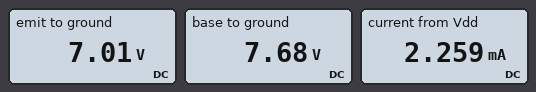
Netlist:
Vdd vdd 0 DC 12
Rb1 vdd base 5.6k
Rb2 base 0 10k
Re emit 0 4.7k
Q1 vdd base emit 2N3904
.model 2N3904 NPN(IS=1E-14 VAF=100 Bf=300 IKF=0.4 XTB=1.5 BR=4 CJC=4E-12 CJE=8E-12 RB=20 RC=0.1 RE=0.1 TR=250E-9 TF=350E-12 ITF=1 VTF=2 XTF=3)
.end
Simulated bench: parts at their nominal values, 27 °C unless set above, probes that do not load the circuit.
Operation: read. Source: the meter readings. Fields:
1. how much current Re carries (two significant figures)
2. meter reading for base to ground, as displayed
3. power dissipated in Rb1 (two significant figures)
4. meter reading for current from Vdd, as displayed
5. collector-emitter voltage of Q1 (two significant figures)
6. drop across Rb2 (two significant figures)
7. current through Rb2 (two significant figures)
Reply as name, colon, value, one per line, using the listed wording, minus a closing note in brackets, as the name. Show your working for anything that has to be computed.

how much current Re carries: (7.01 V) / 4.7 kΩ = 1.5 mA
meter reading for base to ground, as displayed: 7.68 V
power dissipated in Rb1: (12 V - 7.68 V)^2 / 5.6 kΩ = 3.3 mW
meter reading for current from Vdd, as displayed: 2.259 mA
collector-emitter voltage of Q1: 12 V - 7.01 V = 5.0 V
drop across Rb2: 7.68 V = 7.7 V
current through Rb2: (7.68 V) / 10 kΩ = 770 µA
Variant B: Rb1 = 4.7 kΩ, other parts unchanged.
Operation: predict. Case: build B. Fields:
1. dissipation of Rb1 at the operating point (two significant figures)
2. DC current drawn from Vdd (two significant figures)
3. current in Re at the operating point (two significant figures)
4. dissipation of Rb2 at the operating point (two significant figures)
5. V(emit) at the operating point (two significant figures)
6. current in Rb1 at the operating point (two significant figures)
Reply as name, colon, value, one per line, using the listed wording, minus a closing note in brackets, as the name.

dissipation of Rb1 at the operating point: 3.2 mW
DC current drawn from Vdd: 2.4 mA
current in Re at the operating point: 1.6 mA
dissipation of Rb2 at the operating point: 6.6 mW
V(emit) at the operating point: 7.5 V
current in Rb1 at the operating point: 820 µA
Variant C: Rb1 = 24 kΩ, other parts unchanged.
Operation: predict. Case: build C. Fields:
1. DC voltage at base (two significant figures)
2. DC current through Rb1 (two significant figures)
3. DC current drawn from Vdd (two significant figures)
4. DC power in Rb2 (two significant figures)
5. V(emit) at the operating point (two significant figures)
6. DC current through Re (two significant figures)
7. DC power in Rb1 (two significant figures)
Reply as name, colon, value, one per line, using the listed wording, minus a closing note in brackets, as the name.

DC voltage at base: 3.5 V
DC current through Rb1: 350 µA
DC current drawn from Vdd: 960 µA
DC power in Rb2: 1.2 mW
V(emit) at the operating point: 2.9 V
DC current through Re: 610 µA
DC power in Rb1: 3.0 mW
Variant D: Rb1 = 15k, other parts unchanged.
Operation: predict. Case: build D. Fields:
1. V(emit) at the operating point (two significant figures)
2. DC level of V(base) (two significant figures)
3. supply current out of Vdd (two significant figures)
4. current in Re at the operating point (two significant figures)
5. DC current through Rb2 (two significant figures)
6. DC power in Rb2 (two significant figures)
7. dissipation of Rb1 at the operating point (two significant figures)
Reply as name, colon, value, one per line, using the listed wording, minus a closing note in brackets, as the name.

V(emit) at the operating point: 4.1 V
DC level of V(base): 4.8 V
supply current out of Vdd: 1.4 mA
current in Re at the operating point: 880 µA
DC current through Rb2: 480 µA
DC power in Rb2: 2.3 mW
dissipation of Rb1 at the operating point: 3.5 mW
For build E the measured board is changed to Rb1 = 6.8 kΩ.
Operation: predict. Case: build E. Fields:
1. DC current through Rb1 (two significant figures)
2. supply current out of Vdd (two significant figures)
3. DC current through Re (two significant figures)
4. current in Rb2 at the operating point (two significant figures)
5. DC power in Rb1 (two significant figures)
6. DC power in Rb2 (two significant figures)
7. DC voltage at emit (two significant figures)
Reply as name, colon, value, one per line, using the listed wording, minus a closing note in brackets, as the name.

DC current through Rb1: 720 µA
supply current out of Vdd: 2.1 mA
DC current through Re: 1.4 mA
current in Rb2 at the operating point: 710 µA
DC power in Rb1: 3.5 mW
DC power in Rb2: 5.1 mW
DC voltage at emit: 6.5 V
